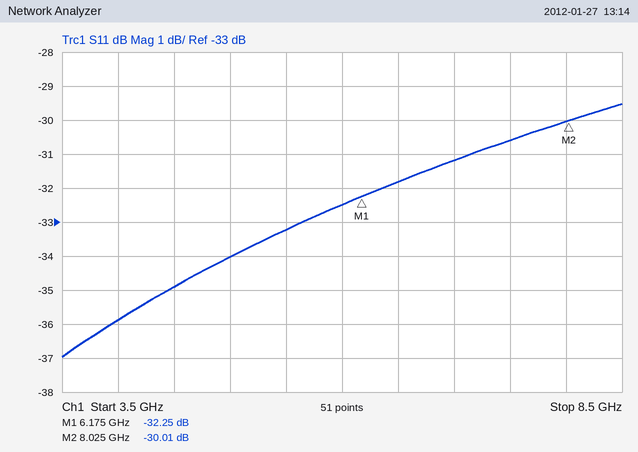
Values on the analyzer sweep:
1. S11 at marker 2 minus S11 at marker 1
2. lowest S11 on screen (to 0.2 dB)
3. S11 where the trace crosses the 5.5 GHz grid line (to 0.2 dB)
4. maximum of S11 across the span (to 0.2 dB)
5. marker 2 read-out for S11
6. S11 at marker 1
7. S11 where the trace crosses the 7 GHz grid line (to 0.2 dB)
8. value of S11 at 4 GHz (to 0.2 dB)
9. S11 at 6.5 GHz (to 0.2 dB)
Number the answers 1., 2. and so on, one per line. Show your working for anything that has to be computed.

1. -30.01 − (-32.25) = 2.24 dB
2. -37.0 dB
3. -33.2 dB
4. -29.6 dB
5. -30.01 dB
6. -32.25 dB
7. -31.2 dB
8. -35.8 dB
9. -31.8 dB
